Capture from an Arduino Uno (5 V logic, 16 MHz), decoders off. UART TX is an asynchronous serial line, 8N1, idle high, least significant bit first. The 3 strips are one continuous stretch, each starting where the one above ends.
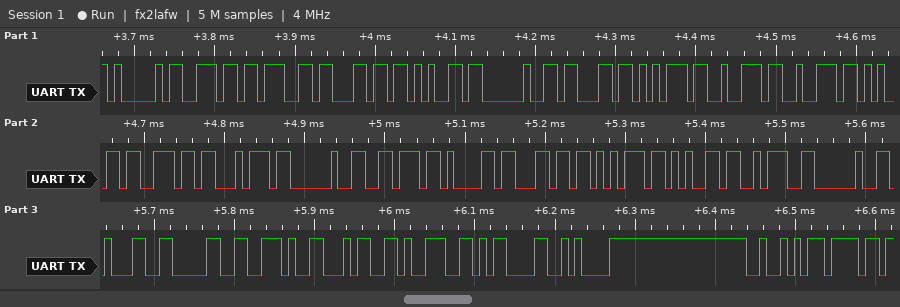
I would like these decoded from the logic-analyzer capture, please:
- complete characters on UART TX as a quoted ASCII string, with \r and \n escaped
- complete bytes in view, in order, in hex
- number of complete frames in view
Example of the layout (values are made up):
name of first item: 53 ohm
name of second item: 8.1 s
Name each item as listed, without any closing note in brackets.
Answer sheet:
complete characters on UART TX as a quoted ASCII string, with \r and \n escaped: "Angle current value: 10.49\r\nRo"
complete bytes in view, in order, in hex: 41 6E 67 6C 65 20 63 75 72 72 65 6E 74 20 76 61 6C 75 65 3A 20 31 30 2E 34 39 0D 0A 52 6F
number of complete frames in view: 30
